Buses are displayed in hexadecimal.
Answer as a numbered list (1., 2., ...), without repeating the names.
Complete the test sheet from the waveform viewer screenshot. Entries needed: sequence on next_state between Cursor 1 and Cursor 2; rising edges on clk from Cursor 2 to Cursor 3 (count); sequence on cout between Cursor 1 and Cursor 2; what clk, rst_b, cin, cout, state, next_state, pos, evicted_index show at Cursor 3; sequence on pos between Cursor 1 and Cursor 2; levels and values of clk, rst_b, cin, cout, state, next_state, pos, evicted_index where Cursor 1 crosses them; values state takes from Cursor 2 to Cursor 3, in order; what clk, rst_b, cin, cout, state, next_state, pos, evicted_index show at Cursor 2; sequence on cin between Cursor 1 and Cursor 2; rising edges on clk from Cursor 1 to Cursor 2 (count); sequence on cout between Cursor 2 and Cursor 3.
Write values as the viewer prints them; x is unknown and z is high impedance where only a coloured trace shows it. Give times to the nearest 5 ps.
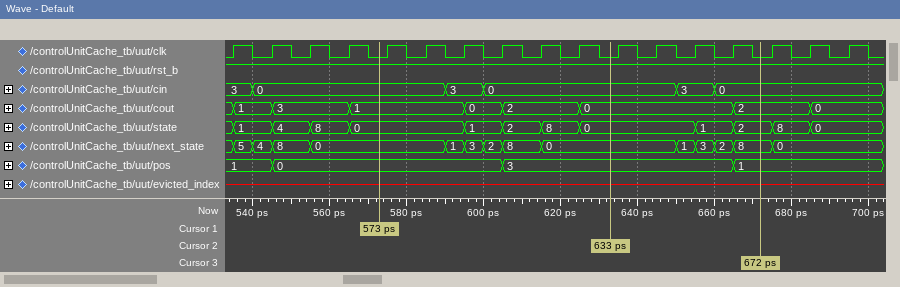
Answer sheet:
1. 0, 1, 3, 2, 8, 0
2. 4
3. 1, 0, 2, 0
4. clk=0, rst_b=1, cin=0, cout=2, state=2, next_state=8, pos=1, evicted_index=x
5. 0, 3
6. clk=0, rst_b=1, cin=0, cout=1, state=0, next_state=0, pos=0, evicted_index=x
7. 0, 1, 2
8. clk=0, rst_b=1, cin=0, cout=0, state=0, next_state=0, pos=3, evicted_index=x
9. 0, 3, 0
10. 6
11. 0, 2
